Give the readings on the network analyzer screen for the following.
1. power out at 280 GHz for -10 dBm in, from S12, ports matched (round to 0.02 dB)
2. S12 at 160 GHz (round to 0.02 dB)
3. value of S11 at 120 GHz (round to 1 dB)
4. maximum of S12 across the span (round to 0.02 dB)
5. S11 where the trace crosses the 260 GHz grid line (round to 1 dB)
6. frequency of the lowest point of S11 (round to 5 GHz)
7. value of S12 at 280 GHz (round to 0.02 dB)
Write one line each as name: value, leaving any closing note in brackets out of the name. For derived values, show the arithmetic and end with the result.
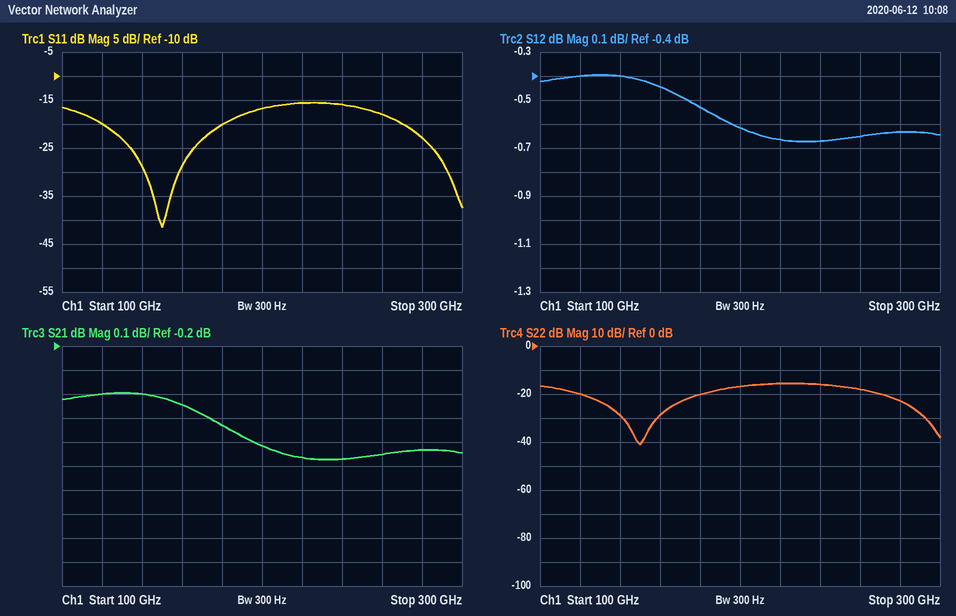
power out at 280 GHz for -10 dBm in, from S12, ports matched: -10 dBm + (-0.64 dB) = -10.64 dBm
S12 at 160 GHz: -0.44 dB
value of S11 at 120 GHz: -20 dB
maximum of S12 across the span: -0.40 dB
S11 where the trace crosses the 260 GHz grid line: -18 dB
frequency of the lowest point of S11: 150 GHz
value of S12 at 280 GHz: -0.64 dB
